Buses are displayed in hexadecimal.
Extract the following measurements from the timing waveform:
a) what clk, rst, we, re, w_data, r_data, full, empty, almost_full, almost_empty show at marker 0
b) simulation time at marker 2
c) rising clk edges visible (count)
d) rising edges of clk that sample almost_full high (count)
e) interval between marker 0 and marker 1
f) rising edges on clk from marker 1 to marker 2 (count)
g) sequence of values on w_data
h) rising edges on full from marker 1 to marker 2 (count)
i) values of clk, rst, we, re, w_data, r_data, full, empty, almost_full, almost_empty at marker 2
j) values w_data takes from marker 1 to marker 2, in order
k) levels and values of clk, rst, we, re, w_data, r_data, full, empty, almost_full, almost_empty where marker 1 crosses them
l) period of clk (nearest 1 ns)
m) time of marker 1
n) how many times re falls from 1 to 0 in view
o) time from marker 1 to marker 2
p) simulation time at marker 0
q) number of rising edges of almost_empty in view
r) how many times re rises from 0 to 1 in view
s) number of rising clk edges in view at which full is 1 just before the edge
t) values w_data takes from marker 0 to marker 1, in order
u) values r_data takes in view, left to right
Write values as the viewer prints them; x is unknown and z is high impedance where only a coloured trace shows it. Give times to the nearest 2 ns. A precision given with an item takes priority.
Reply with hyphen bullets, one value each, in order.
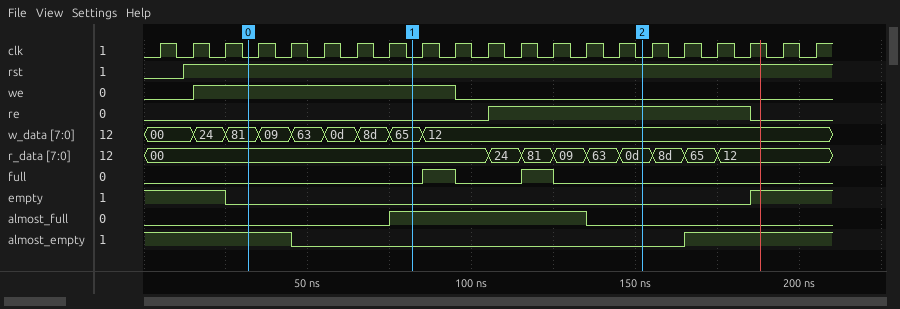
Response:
- clk=0, rst=1, we=1, re=0, w_data=81, r_data=00, full=0, empty=0, almost_full=0, almost_empty=1
- 152 ns
- 21
- 6
- 50 ns
- 7
- 00, 24, 81, 09, 63, 0d, 8d, 65, 12
- 2
- clk=0, rst=1, we=0, re=1, w_data=12, r_data=0d, full=0, empty=0, almost_full=0, almost_empty=0
- 65, 12
- clk=0, rst=1, we=1, re=0, w_data=65, r_data=00, full=0, empty=0, almost_full=1, almost_empty=0
- 10 ns
- 82 ns
- 1
- 70 ns
- 32 ns
- 1
- 1
- 2
- 81, 09, 63, 0d, 8d, 65
- 00, 24, 81, 09, 63, 0d, 8d, 65, 12
